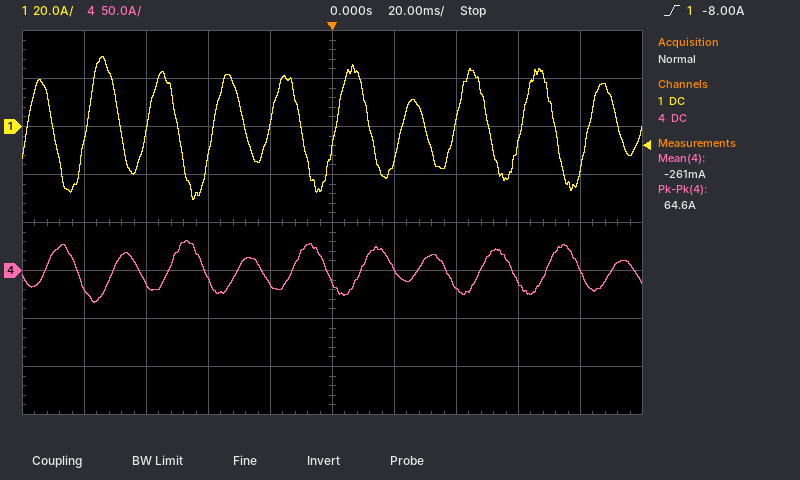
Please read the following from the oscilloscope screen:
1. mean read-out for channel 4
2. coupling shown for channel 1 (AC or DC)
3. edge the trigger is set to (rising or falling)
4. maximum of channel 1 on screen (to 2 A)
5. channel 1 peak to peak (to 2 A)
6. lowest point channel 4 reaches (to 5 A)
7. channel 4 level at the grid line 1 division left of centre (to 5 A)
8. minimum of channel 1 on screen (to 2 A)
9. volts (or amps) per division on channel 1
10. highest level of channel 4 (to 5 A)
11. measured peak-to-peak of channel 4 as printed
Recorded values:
-261 mA
DC
rising
30 A
60 A
-35 A
-15 A
-30 A
20 A
30 A
64.6 A
